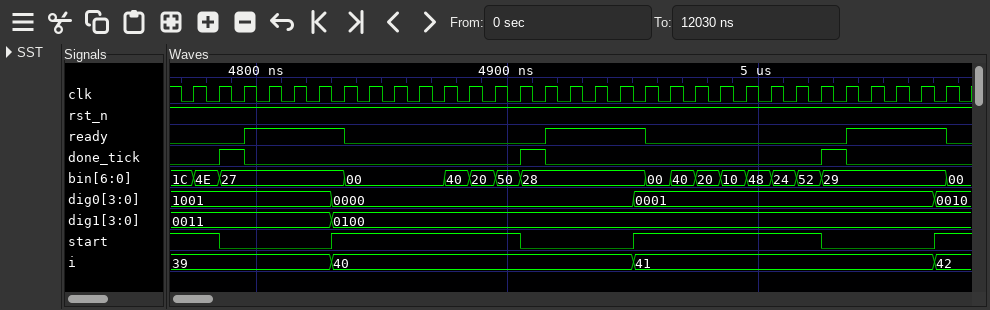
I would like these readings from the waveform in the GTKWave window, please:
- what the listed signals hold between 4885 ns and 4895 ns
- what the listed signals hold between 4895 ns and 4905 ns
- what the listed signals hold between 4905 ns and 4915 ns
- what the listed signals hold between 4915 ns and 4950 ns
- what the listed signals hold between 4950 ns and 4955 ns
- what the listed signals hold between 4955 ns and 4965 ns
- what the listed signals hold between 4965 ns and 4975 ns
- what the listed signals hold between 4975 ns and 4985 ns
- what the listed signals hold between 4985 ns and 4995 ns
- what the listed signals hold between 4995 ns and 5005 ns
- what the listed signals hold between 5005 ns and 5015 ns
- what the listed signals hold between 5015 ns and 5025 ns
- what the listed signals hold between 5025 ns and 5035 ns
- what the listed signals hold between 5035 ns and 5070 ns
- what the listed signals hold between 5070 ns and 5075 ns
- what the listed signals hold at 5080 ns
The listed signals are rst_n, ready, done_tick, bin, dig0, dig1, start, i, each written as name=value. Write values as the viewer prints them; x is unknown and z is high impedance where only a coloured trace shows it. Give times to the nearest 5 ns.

rst_n=1, ready=0, done_tick=0, bin=20, dig0=0000, dig1=0100, start=1, i=40
rst_n=1, ready=0, done_tick=0, bin=50, dig0=0000, dig1=0100, start=1, i=40
rst_n=1, ready=0, done_tick=1, bin=28, dig0=0000, dig1=0100, start=0, i=40
rst_n=1, ready=1, done_tick=0, bin=28, dig0=0000, dig1=0100, start=0, i=40
rst_n=1, ready=1, done_tick=0, bin=28, dig0=0001, dig1=0100, start=1, i=41
rst_n=1, ready=0, done_tick=0, bin=00, dig0=0001, dig1=0100, start=1, i=41
rst_n=1, ready=0, done_tick=0, bin=40, dig0=0001, dig1=0100, start=1, i=41
rst_n=1, ready=0, done_tick=0, bin=20, dig0=0001, dig1=0100, start=1, i=41
rst_n=1, ready=0, done_tick=0, bin=10, dig0=0001, dig1=0100, start=1, i=41
rst_n=1, ready=0, done_tick=0, bin=48, dig0=0001, dig1=0100, start=1, i=41
rst_n=1, ready=0, done_tick=0, bin=24, dig0=0001, dig1=0100, start=1, i=41
rst_n=1, ready=0, done_tick=0, bin=52, dig0=0001, dig1=0100, start=1, i=41
rst_n=1, ready=0, done_tick=1, bin=29, dig0=0001, dig1=0100, start=0, i=41
rst_n=1, ready=1, done_tick=0, bin=29, dig0=0001, dig1=0100, start=0, i=41
rst_n=1, ready=1, done_tick=0, bin=29, dig0=0010, dig1=0100, start=1, i=42
rst_n=1, ready=0, done_tick=0, bin=00, dig0=0010, dig1=0100, start=1, i=42
